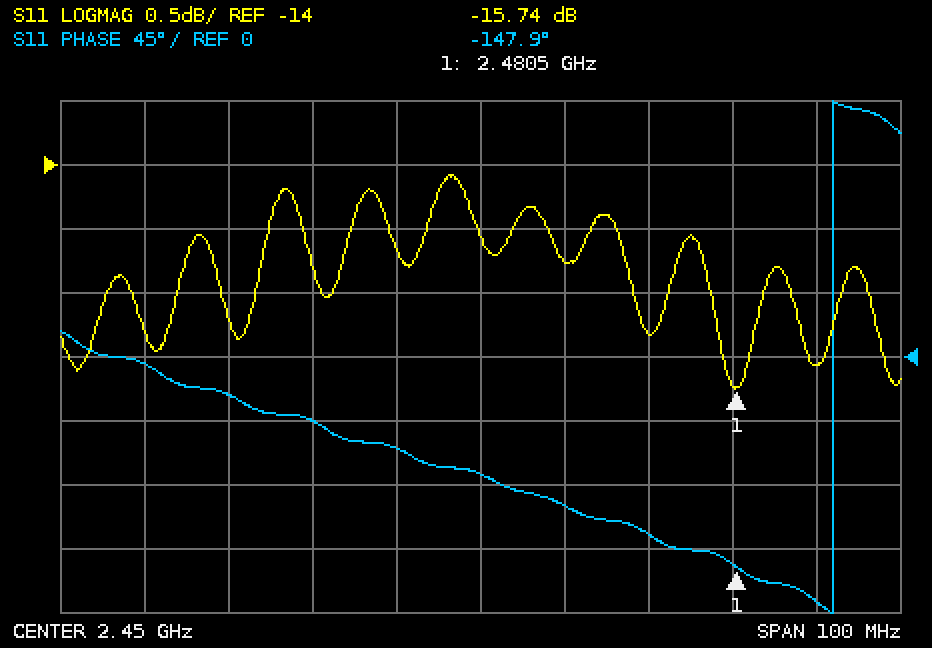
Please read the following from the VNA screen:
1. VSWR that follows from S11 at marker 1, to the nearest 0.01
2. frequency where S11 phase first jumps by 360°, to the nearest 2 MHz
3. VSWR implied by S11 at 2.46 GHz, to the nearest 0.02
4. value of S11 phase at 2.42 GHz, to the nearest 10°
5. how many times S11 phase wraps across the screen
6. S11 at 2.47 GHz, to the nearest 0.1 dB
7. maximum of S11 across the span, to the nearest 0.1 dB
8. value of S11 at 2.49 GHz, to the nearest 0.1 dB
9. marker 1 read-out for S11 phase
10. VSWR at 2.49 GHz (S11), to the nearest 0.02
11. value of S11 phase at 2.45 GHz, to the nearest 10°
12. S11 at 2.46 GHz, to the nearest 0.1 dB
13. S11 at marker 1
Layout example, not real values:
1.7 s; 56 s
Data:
1.39; 2.492 GHz; 1.44; -30°; 1; -15.3 dB; -14.1 dB; -15.6 dB; -147.9°; 1.40; -80°; -14.8 dB; -15.74 dB
